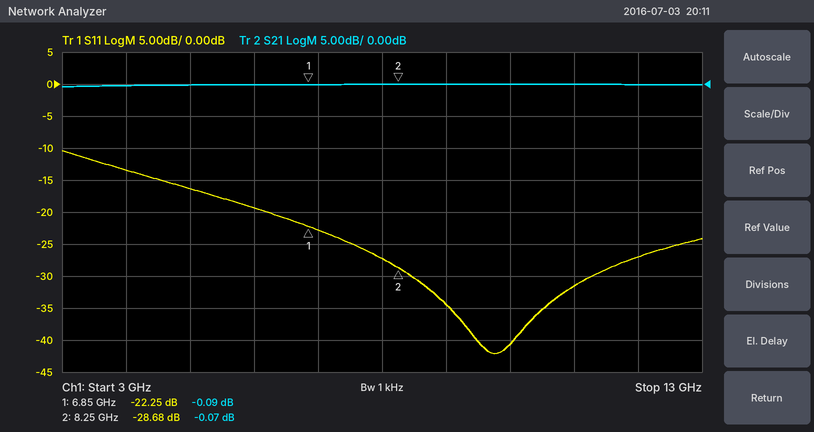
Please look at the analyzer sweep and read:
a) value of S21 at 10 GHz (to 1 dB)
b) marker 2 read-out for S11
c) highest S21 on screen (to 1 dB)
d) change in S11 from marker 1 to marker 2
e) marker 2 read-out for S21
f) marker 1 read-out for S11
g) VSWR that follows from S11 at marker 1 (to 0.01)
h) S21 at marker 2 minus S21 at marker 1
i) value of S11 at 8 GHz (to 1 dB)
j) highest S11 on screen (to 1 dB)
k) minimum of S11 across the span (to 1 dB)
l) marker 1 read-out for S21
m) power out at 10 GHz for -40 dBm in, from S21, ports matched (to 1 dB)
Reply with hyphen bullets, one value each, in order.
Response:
- 0 dB
- -28.68 dB
- 0 dB
- -6.43 dB
- -0.07 dB
- -22.25 dB
- 1.17
- 0.02 dB
- -27 dB
- -10 dB
- -42 dB
- -0.09 dB
- -40 dBm
